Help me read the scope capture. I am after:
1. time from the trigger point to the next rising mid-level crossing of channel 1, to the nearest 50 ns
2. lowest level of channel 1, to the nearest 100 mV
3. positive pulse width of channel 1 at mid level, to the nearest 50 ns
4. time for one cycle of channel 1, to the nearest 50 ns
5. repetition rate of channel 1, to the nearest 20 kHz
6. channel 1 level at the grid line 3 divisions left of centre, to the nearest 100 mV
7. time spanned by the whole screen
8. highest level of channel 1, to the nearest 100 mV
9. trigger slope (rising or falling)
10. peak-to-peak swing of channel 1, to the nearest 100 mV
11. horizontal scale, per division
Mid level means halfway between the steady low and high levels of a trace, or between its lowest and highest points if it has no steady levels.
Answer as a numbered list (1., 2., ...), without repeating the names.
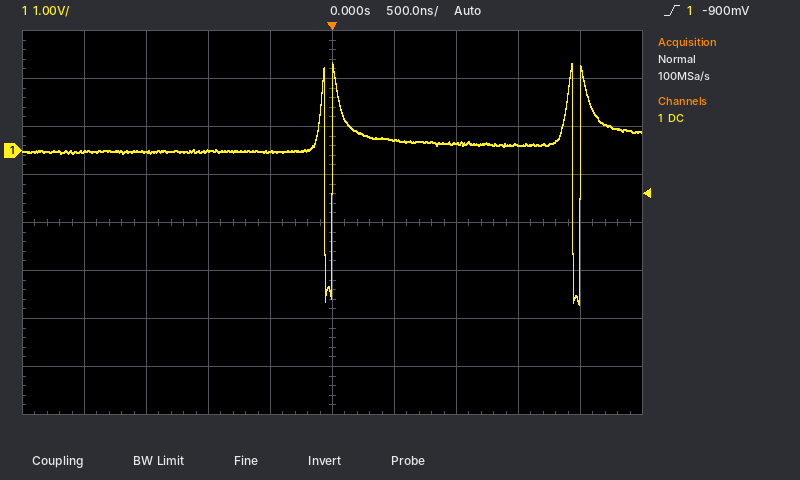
1. 2.00 µs
2. -3.2 V
3. 1.95 µs
4. 2.00 µs
5. 500 kHz
6. 0.0 V
7. 5 µs
8. 1.8 V
9. rising
10. 5.0 V
11. 500 ns
